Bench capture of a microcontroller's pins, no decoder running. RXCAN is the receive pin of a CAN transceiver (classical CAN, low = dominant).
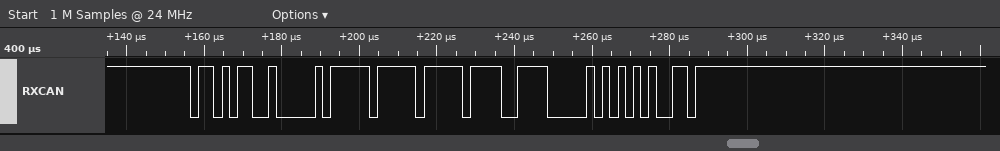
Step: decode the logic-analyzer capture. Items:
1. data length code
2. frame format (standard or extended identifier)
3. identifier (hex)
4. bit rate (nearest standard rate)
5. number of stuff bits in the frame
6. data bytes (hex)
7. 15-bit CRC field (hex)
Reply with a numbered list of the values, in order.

1. 3
2. standard
3. 0x6B2
4. 500 kbit/s
5. 5
6. FF FF 9E
7. 0x02A9
